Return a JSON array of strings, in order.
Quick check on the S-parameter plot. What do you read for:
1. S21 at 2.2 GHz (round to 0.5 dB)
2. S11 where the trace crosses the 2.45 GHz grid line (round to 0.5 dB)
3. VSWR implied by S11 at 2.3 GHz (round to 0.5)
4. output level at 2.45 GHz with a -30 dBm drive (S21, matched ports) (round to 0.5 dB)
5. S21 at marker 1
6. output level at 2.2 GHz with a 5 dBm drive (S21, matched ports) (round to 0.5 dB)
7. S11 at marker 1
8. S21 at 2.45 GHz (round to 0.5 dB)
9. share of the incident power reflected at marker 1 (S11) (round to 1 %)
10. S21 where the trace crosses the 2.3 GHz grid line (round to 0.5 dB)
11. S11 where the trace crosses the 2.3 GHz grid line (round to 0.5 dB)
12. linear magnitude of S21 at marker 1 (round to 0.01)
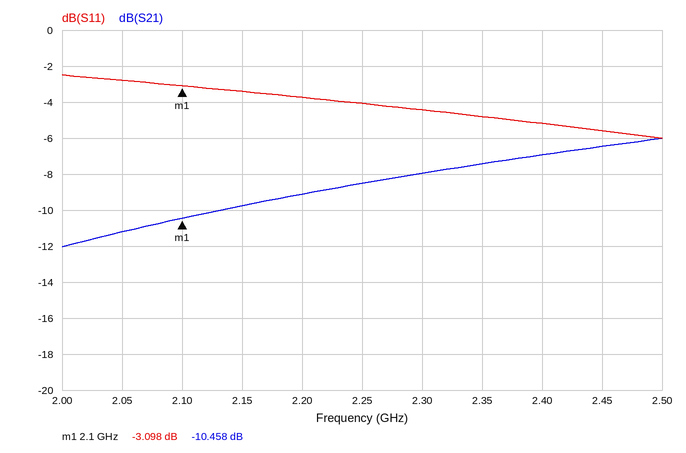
["-9.0 dB", "-5.5 dB", "4.0", "-36.5 dBm", "-10.458 dB", "-4.0 dBm", "-3.098 dB", "-6.5 dB", "49 %", "-8.0 dB", "-4.5 dB", "0.30"]
